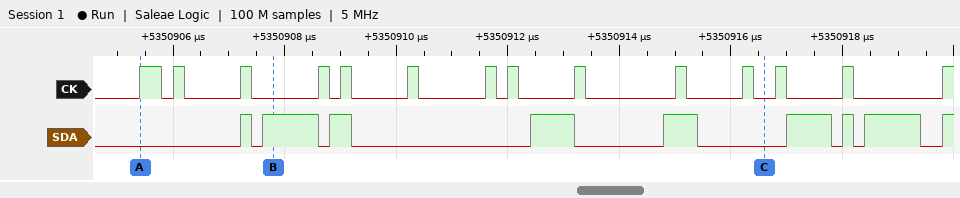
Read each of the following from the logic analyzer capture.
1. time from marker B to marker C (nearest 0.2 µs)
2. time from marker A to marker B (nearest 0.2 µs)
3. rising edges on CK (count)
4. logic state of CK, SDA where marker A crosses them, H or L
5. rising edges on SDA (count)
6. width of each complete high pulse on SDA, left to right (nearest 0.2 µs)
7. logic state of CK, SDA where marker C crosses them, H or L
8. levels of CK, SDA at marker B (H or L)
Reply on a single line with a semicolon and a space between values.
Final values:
8.8 µs; 2.4 µs; 14; CK=H, SDA=L; 9; 0.2 µs, 1 µs, 0.4 µs, 0.8 µs, 0.6 µs, 0.8 µs, 0.2 µs, 1 µs; CK=L, SDA=L; CK=L, SDA=H
